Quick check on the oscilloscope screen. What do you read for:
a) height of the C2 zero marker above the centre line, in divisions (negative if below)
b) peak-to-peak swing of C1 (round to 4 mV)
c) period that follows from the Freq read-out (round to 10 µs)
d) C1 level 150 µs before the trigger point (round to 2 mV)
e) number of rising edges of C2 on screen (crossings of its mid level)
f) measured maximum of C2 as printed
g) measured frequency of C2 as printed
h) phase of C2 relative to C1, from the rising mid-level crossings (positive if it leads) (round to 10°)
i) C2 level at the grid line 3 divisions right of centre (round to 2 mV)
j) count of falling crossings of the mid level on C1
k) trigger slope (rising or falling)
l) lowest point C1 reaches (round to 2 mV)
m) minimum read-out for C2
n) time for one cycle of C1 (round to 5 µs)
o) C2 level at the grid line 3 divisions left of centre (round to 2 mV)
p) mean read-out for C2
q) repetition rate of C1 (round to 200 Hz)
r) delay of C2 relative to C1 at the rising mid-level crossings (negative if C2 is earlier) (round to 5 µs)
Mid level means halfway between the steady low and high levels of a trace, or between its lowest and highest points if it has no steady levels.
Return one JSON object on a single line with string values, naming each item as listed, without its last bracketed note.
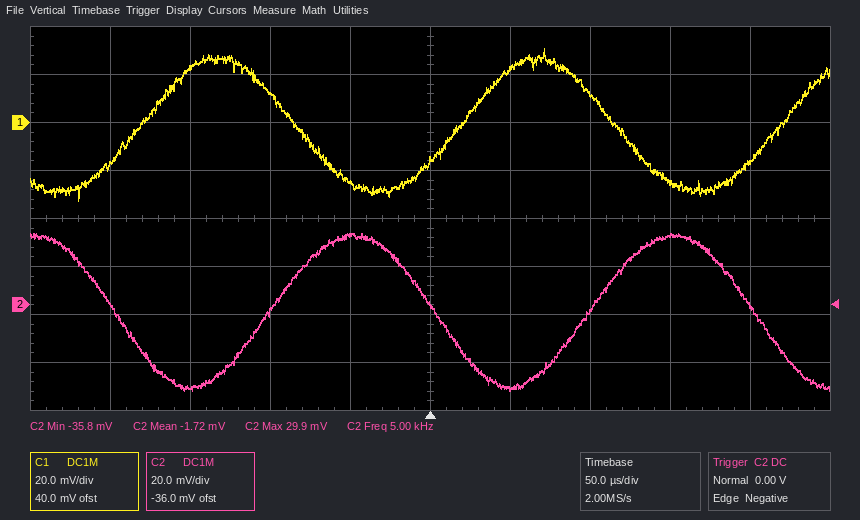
{"height of the C2 zero marker above the centre line, in divisions": "-1.8 div", "peak-to-peak swing of C1": "64 mV", "period that follows from the Freq read-out": "200 µs", "C1 level 150 µs before the trigger point": "22 mV", "number of rising edges of C2 on screen": "2", "measured maximum of C2 as printed": "29.9 mV", "measured frequency of C2 as printed": "5.00 kHz", "phase of C2 relative to C1, from the rising mid-level crossings (positive if it leads)": "-140°", "C2 level at the grid line 3 divisions right of centre": "30 mV", "count of falling crossings of the mid level on C1": "2", "trigger slope": "falling", "lowest point C1 reaches": "-32 mV", "minimum read-out for C2": "-35.8 mV", "time for one cycle of C1": "200 µs", "C2 level at the grid line 3 divisions left of centre": "-34 mV", "mean read-out for C2": "-1.72 mV", "repetition rate of C1": "5.0 kHz", "delay of C2 relative to C1 at the rising mid-level crossings (negative if C2 is earlier)": "+80 µs"}
